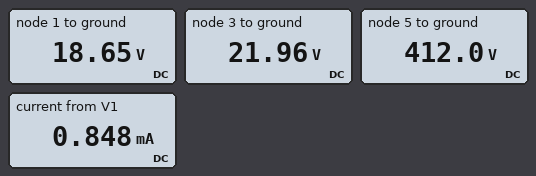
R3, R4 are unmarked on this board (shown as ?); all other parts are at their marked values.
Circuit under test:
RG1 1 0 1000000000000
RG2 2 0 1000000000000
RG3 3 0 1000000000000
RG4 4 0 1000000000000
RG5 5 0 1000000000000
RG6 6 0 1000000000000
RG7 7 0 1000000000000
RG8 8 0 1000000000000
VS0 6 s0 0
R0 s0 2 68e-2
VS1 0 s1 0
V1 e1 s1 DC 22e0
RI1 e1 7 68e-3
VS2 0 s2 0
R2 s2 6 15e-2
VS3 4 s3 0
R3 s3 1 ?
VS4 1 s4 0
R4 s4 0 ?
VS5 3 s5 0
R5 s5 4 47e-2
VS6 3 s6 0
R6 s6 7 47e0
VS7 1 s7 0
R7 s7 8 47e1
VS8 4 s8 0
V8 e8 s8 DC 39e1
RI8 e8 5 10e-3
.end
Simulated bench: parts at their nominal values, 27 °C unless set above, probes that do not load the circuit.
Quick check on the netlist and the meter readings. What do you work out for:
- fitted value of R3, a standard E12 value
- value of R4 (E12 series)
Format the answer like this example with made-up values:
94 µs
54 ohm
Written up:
3.9 kΩ
22 kΩ
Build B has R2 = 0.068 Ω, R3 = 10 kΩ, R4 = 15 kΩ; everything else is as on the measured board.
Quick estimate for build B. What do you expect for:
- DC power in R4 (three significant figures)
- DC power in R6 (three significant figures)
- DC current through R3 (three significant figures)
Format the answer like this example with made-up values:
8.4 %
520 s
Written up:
11.6 mW
36.3 µW
878 µA
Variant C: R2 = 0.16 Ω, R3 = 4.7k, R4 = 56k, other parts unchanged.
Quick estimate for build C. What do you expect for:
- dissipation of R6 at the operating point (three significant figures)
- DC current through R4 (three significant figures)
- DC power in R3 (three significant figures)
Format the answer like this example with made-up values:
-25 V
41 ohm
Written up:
6.16 µW
362 µA
616 µW
